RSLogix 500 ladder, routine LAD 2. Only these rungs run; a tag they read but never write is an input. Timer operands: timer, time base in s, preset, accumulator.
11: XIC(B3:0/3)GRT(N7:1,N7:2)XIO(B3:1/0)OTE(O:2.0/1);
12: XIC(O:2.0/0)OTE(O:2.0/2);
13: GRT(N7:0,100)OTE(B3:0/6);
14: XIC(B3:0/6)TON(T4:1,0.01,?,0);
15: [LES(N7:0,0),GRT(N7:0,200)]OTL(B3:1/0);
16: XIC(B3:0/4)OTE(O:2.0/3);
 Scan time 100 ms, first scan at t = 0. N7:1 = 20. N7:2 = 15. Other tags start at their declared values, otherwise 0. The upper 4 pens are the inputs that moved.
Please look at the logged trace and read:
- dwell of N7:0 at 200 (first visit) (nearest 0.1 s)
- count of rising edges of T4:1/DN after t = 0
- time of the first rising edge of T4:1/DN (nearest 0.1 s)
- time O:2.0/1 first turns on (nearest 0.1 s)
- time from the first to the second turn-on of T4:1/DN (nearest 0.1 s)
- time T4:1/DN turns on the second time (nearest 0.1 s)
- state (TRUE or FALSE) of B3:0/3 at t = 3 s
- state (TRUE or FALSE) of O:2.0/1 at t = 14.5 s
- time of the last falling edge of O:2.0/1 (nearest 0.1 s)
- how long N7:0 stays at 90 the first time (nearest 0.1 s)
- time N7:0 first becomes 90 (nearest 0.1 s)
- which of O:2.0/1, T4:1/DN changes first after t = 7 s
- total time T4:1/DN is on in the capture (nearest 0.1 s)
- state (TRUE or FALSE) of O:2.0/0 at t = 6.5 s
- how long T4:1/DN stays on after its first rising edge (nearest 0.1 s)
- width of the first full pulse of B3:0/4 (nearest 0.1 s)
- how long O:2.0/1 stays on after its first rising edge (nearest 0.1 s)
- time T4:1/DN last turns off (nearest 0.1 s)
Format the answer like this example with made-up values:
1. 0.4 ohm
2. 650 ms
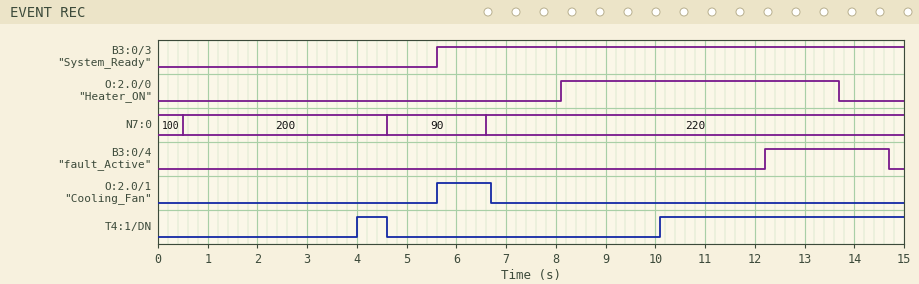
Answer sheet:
1. 4.1 s
2. 2
3. 4.0 s
4. 5.6 s
5. 6.1 s
6. 10.1 s
7. FALSE
8. FALSE
9. 6.7 s
10. 2.0 s
11. 4.6 s
12. T4:1/DN
13. 5.5 s
14. FALSE
15. 0.6 s
16. 2.5 s
17. 1.1 s
18. 4.6 s
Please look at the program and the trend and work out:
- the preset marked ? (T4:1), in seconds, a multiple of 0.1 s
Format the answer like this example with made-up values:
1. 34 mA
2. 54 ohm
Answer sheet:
1. 3.5 s
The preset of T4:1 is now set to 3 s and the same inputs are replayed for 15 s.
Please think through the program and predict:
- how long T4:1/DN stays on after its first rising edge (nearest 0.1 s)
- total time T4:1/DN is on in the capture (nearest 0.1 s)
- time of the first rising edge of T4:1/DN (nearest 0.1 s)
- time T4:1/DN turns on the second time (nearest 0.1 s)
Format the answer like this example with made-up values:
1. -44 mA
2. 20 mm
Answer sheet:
1. 1.1 s
2. 6.5 s
3. 3.5 s
4. 9.6 s
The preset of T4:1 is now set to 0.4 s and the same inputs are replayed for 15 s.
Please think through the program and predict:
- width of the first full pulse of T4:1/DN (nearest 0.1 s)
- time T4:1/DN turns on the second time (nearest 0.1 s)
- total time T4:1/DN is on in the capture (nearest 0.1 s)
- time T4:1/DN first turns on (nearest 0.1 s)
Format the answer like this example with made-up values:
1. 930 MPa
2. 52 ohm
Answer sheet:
1. 3.7 s
2. 7.0 s
3. 11.7 s
4. 0.9 s
